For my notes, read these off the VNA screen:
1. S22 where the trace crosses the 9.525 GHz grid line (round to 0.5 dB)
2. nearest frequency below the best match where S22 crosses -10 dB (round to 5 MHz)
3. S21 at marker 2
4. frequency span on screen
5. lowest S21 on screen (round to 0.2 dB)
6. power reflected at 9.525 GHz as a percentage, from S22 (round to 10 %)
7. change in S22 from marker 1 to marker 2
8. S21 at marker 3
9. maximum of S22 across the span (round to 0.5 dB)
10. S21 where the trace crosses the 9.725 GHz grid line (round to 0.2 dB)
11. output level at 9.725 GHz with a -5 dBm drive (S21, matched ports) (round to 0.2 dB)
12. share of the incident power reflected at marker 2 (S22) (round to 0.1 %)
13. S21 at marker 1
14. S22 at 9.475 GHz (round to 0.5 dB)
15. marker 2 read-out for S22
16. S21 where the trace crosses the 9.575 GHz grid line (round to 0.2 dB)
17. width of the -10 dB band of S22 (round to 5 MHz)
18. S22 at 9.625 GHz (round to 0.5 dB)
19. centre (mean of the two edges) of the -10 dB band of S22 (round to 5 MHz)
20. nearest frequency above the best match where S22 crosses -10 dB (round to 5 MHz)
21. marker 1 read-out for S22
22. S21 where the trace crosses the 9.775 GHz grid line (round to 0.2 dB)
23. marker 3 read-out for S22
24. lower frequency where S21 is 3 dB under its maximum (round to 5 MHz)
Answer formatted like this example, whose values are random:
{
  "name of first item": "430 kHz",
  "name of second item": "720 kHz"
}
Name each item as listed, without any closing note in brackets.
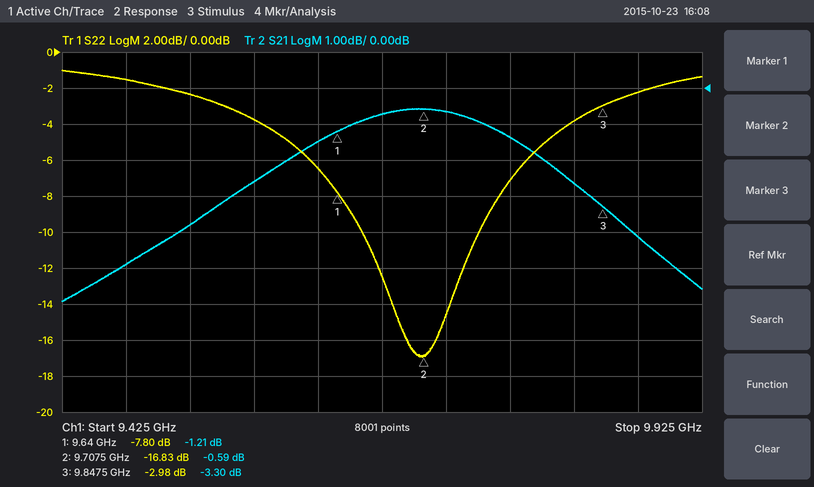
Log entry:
{
  "S22 where the trace crosses the 9.525 GHz grid line": "-2.5 dB",
  "nearest frequency below the best match where S22 crosses -10 dB": "9.660 GHz",
  "S21 at marker 2": "-0.59 dB",
  "frequency span on screen": "500 MHz",
  "lowest S21 on screen": "-6.0 dB",
  "power reflected at 9.525 GHz as a percentage, from S22": "60 %",
  "change in S22 from marker 1 to marker 2": "-9.03 dB",
  "S21 at marker 3": "-3.30 dB",
  "maximum of S22 across the span": "-1.0 dB",
  "S21 where the trace crosses the 9.725 GHz grid line": "-0.6 dB",
  "output level at 9.725 GHz with a -5 dBm drive (S21, matched ports)": "-5.6 dBm",
  "share of the incident power reflected at marker 2 (S22)": "2.1 %",
  "S21 at marker 1": "-1.21 dB",
  "S22 at 9.475 GHz": "-1.5 dB",
  "marker 2 read-out for S22": "-16.83 dB",
  "S21 where the trace crosses the 9.575 GHz grid line": "-2.6 dB",
  "width of the -10 dB band of S22": "90 MHz",
  "S22 at 9.625 GHz": "-6.5 dB",
  "centre (mean of the two edges) of the -10 dB band of S22": "9.705 GHz",
  "nearest frequency above the best match where S22 crosses -10 dB": "9.750 GHz",
  "marker 1 read-out for S22": "-7.80 dB",
  "S21 where the trace crosses the 9.775 GHz grid line": "-1.4 dB",
  "marker 3 read-out for S22": "-2.98 dB",
  "lower frequency where S21 is 3 dB under its maximum": "9.535 GHz"
}
